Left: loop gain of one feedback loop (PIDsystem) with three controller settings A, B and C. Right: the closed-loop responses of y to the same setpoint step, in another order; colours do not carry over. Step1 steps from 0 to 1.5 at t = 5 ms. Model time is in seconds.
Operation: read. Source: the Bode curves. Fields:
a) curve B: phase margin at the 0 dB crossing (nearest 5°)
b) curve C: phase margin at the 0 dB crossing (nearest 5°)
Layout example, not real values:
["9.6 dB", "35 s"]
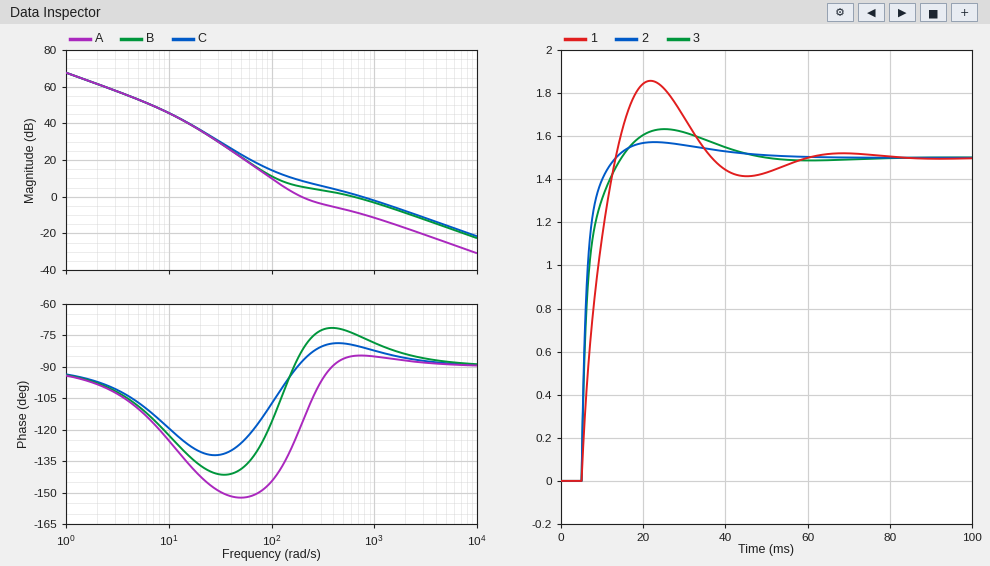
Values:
["105°", "100°"]
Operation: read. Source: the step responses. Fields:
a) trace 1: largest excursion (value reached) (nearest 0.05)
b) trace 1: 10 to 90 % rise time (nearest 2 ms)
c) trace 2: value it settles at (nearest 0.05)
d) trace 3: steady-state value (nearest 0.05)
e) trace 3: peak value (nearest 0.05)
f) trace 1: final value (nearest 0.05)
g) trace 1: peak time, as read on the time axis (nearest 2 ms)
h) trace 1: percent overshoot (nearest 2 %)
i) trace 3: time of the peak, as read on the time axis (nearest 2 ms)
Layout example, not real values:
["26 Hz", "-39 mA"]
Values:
["1.85", "6 ms", "1.50", "1.50", "1.65", "1.50", "22 ms", "24 %", "26 ms"]
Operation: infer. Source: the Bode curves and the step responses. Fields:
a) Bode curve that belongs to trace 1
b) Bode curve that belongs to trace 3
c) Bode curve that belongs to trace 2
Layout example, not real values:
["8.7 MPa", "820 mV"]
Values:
["A", "B", "C"]
